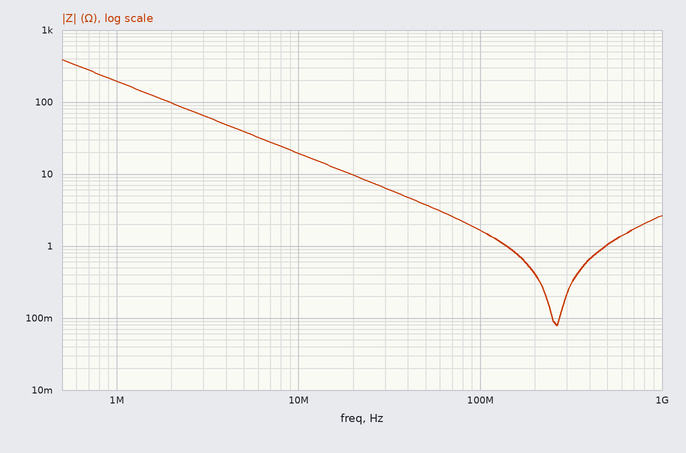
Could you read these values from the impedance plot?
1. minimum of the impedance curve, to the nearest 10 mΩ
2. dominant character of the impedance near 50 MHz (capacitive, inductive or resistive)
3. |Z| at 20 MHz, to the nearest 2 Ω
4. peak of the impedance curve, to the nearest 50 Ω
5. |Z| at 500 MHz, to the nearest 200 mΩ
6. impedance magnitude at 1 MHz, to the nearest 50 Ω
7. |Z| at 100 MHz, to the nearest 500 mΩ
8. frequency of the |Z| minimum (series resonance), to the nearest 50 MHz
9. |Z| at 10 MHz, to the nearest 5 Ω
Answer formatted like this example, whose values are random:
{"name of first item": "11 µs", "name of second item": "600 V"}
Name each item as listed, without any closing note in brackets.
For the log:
{"minimum of the impedance curve, to the nearest 10 mΩ": "80 mΩ", "dominant character of the impedance near 50 MHz": "capacitive", "|Z| at 20 MHz, to the nearest 2 Ω": "10 Ω", "peak of the impedance curve, to the nearest 50 Ω": "400 Ω", "|Z| at 500 MHz, to the nearest 200 mΩ": "1.0 Ω", "impedance magnitude at 1 MHz, to the nearest 50 Ω": "200 Ω", "|Z| at 100 MHz, to the nearest 500 mΩ": "1.5 Ω", "frequency of the |Z| minimum (series resonance), to the nearest 50 MHz": "250 MHz", "|Z| at 10 MHz, to the nearest 5 Ω": "20 Ω"}
